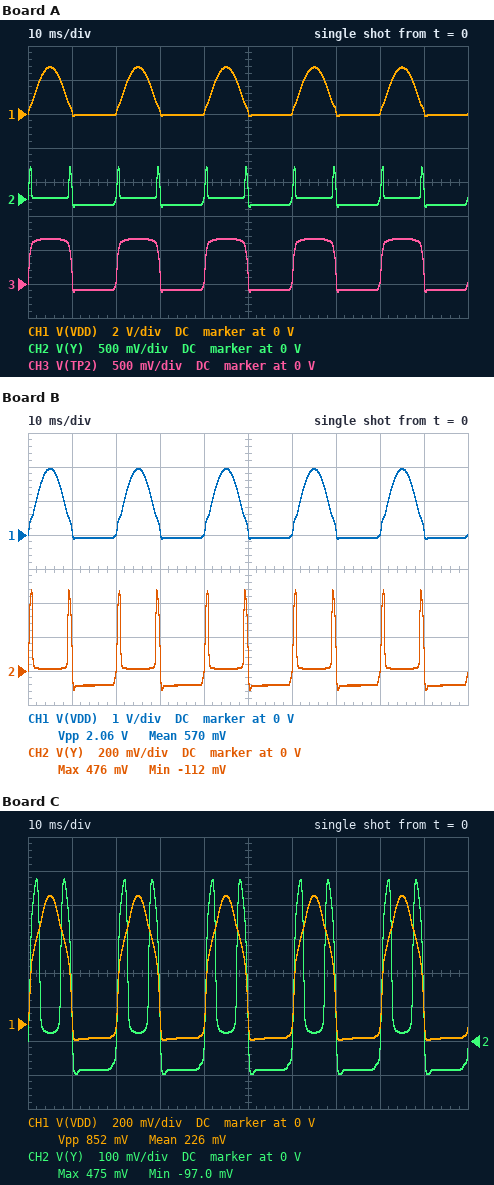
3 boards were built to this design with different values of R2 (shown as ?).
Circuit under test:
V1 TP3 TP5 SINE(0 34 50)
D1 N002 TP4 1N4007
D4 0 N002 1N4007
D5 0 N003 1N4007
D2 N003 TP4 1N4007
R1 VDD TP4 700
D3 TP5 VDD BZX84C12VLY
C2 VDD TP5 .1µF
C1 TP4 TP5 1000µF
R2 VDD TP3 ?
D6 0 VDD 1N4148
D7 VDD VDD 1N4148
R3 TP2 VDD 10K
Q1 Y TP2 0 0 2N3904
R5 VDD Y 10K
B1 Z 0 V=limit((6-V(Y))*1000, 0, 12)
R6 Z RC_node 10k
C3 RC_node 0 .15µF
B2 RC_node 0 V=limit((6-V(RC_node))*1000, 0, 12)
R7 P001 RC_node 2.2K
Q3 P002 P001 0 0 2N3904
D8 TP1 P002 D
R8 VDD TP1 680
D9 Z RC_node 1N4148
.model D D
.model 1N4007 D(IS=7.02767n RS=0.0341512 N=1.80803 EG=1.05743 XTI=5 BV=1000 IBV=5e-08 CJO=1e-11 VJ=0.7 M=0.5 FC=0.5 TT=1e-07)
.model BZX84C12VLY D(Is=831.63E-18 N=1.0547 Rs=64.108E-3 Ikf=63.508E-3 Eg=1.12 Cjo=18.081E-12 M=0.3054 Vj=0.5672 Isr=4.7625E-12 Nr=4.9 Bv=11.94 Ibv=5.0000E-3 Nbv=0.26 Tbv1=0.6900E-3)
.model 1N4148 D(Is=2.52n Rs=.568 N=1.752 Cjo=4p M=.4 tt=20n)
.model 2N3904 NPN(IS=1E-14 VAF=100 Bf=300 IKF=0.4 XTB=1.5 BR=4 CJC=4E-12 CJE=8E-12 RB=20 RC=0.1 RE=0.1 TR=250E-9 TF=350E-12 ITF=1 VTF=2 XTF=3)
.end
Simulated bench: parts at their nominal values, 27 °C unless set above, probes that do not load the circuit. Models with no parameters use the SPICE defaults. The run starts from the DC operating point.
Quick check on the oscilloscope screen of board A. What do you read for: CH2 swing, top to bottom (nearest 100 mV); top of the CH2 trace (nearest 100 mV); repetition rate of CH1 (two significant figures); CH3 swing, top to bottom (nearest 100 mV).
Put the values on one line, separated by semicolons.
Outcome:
600 mV; 500 mV; 50 Hz; 800 mV
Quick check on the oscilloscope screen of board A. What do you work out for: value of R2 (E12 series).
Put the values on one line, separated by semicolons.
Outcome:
3.3 kΩ
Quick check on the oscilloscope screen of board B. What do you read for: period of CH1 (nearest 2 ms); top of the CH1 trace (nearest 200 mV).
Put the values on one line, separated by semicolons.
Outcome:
20 ms; 2.0 V
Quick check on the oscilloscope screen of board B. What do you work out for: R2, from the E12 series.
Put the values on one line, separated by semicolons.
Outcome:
4.7 kΩ
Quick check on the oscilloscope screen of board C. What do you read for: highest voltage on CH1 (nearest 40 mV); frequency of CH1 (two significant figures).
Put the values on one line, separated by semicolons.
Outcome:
760 mV; 50 Hz
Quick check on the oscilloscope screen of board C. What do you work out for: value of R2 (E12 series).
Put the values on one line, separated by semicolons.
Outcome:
12 kΩ
